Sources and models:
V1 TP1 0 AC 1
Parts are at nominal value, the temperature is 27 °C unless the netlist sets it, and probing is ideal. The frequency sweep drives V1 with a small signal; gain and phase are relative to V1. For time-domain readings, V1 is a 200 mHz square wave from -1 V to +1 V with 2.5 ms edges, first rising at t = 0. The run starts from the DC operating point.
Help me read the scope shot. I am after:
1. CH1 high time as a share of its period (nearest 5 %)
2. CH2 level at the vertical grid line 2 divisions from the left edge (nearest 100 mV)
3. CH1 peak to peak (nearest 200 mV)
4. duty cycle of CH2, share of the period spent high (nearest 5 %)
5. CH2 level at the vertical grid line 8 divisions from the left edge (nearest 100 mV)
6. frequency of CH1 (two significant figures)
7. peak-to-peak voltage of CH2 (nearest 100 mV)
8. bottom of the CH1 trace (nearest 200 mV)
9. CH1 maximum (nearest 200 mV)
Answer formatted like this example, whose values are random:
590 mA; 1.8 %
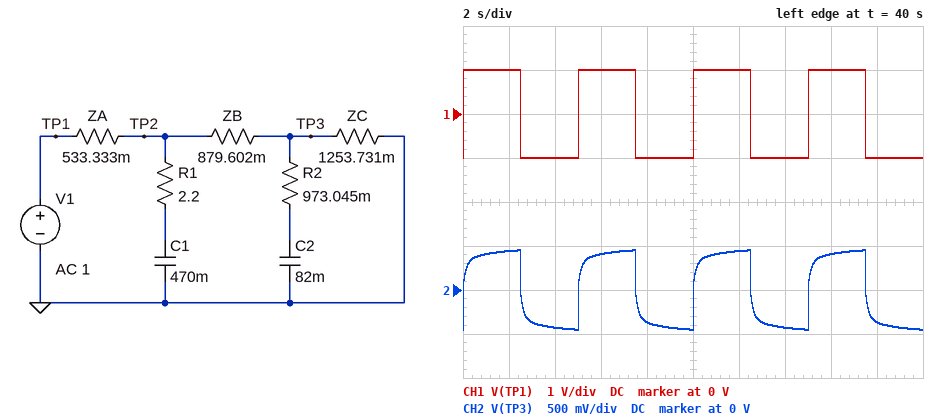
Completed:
50 %; -400 mV; 2.0 V; 50 %; 400 mV; 200 mHz; 900 mV; -1.0 V; 1.0 V
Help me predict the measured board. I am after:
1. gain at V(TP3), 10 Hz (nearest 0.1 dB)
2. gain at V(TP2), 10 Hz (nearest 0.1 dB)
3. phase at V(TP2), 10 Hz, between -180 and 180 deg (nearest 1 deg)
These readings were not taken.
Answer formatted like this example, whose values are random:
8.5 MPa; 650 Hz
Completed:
-12.4 dB; -4.2 dB; -1 deg
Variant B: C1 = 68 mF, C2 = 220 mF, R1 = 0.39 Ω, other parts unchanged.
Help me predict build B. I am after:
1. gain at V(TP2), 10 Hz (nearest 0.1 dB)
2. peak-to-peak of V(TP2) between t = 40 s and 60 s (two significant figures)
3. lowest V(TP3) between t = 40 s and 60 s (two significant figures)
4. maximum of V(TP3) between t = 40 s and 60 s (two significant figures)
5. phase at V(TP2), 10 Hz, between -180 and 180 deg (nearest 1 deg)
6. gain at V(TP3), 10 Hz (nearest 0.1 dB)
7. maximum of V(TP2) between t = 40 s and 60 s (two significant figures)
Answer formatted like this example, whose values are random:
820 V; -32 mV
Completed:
-7.8 dB; 1.6 V; -470 mV; 470 mV; -14 deg; -16.1 dB; 800 mV
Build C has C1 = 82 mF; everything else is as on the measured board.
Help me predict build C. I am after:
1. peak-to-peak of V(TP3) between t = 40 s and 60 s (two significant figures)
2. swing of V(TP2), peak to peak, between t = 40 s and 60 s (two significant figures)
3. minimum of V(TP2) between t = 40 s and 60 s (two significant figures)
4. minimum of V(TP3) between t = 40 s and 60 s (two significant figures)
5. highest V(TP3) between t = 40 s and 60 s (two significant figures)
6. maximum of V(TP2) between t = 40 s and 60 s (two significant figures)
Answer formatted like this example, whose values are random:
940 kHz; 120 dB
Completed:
940 mV; 1.6 V; -800 mV; -470 mV; 470 mV; 800 mV
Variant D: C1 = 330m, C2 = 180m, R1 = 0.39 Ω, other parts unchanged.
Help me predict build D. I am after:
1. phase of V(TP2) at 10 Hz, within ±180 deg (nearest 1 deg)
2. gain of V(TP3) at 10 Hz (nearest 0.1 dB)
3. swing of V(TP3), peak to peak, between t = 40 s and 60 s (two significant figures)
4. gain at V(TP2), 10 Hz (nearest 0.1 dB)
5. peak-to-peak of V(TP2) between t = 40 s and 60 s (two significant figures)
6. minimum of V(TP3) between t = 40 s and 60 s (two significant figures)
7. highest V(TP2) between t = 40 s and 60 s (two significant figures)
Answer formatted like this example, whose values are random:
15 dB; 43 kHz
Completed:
-4 deg; -17.0 dB; 940 mV; -8.7 dB; 1.6 V; -470 mV; 800 mV
